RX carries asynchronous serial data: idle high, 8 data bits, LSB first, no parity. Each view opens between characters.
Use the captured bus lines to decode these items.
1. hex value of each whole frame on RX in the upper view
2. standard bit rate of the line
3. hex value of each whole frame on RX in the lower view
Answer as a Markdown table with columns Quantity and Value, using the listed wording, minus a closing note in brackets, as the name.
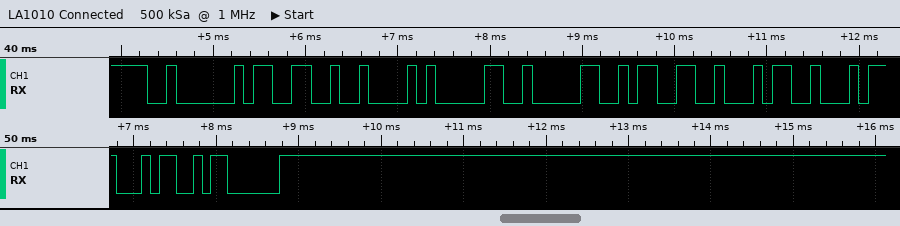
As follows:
| Quantity | Value |
|---|---|
| hex value of each whole frame on RX in the upper view | 02, 33, 42, 30, 30, 33, 34 |
| standard bit rate of the line | 9600 baud |
| hex value of each whole frame on RX in the lower view | 34, 03 |
